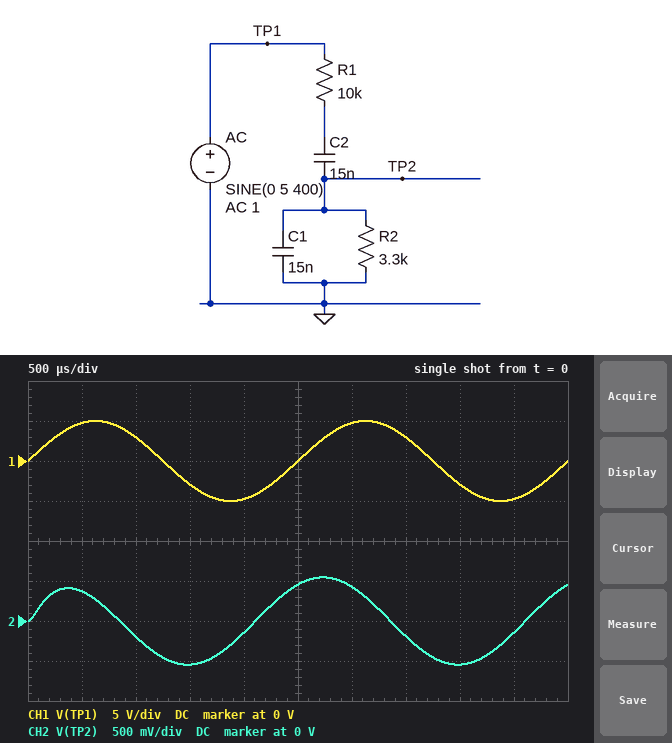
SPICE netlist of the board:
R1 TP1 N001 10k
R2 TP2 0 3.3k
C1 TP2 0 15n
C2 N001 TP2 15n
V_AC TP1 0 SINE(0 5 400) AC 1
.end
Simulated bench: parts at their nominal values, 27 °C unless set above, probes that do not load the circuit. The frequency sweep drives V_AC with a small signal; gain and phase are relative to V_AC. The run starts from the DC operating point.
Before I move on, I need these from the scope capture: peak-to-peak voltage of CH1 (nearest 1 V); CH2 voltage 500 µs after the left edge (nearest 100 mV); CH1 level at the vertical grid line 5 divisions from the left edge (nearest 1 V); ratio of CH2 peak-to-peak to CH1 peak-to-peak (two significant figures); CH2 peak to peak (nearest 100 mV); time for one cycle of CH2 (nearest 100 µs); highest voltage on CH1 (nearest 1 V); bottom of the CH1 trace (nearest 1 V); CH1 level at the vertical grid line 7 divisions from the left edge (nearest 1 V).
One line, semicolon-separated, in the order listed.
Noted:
10 V; 400 mV; 0 V; 0.11; 1.1 V; 2.5 ms; 5 V; -5 V; 3 V
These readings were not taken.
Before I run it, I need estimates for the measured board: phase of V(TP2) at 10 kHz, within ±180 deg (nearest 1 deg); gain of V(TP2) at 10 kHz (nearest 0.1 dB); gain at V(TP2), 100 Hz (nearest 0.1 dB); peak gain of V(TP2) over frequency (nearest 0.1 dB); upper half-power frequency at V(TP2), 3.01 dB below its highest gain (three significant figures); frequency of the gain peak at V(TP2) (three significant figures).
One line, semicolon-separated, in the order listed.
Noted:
-61 deg; -20.3 dB; -30.2 dB; -14.0 dB; 5.91 kHz; 1.85 kHz
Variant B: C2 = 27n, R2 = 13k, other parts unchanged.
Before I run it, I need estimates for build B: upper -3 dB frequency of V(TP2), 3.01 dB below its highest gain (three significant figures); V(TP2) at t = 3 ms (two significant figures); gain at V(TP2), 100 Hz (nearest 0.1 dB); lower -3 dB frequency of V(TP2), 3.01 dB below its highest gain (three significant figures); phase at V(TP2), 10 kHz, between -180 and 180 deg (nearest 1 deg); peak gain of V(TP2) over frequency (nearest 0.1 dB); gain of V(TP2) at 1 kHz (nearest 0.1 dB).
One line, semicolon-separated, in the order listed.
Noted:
2.65 kHz; 2.0 V; -14.0 dB; 182 Hz; -76 deg; -7.3 dB; -7.5 dB
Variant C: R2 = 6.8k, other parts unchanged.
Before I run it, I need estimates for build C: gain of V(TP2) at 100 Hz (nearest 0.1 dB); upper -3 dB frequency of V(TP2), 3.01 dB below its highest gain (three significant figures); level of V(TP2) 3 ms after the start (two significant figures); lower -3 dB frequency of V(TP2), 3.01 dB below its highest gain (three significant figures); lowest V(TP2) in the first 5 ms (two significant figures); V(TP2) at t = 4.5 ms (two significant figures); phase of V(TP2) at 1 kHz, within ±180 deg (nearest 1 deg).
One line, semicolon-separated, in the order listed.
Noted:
-24.0 dB; 4.09 kHz; 900 mV; 405 Hz; -1.0 V; -450 mV; 10 deg
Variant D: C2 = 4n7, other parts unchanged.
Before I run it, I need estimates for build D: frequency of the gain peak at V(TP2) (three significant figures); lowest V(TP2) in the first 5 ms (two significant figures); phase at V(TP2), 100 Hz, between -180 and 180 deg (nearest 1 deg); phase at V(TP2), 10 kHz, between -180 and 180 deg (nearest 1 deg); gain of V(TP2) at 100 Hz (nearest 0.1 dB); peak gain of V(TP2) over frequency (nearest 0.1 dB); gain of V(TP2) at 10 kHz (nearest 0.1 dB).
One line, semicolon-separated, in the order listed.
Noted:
3.30 kHz; -190 mV; 86 deg; -49 deg; -40.2 dB; -17.2 dB; -20.9 dB
